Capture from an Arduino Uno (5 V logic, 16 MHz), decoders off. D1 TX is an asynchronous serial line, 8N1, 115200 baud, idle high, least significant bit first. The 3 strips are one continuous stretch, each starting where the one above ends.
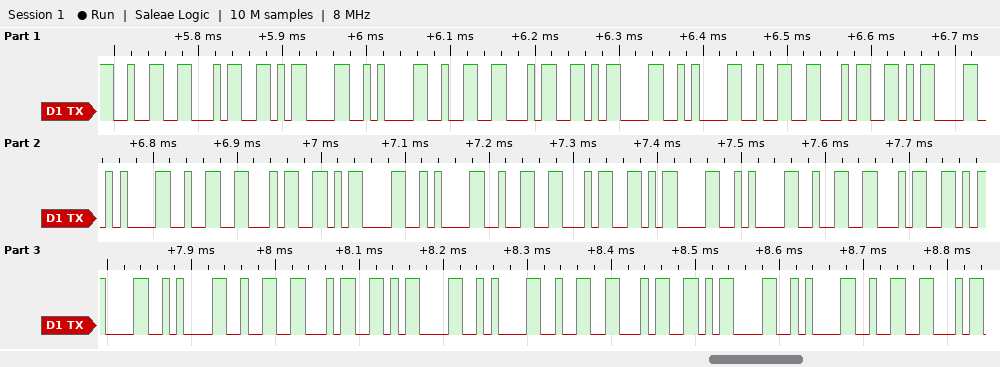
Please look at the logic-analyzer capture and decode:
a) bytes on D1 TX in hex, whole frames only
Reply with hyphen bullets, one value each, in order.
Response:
- 32 34 0D 0A 32 34 0D 0A 32 34 0D 0A 32 34 0D 0A 32 34 0D 0A 32 34 0D 0A 32 34 0D 0A 32 34 0D 0A 32
